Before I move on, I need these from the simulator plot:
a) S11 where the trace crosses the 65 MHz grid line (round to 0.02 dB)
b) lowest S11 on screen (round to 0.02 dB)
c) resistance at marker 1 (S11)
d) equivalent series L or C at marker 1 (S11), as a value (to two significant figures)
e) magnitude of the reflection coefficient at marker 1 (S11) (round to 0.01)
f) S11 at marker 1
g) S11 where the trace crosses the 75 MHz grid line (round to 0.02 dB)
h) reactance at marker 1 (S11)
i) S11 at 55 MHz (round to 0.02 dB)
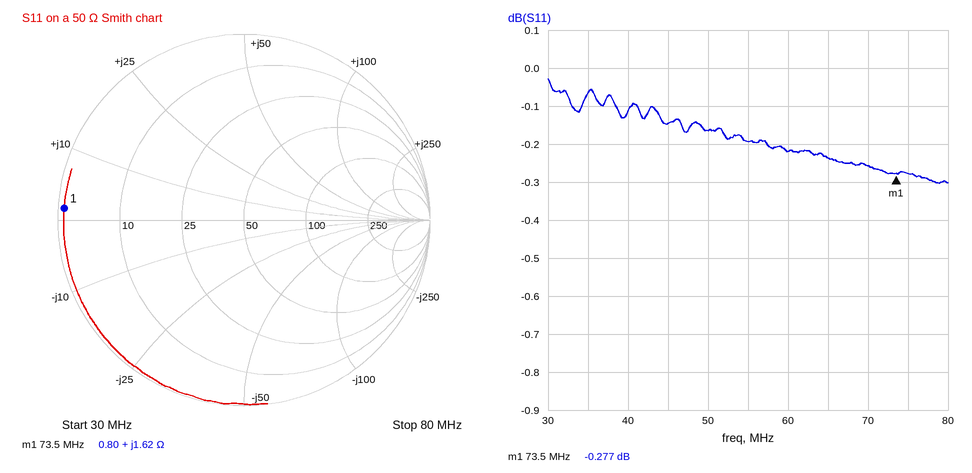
-0.24 dB
-0.30 dB
0.80 Ω
3.5 nH
0.97
-0.277 dB
-0.28 dB
+1.62 Ω
-0.20 dB
